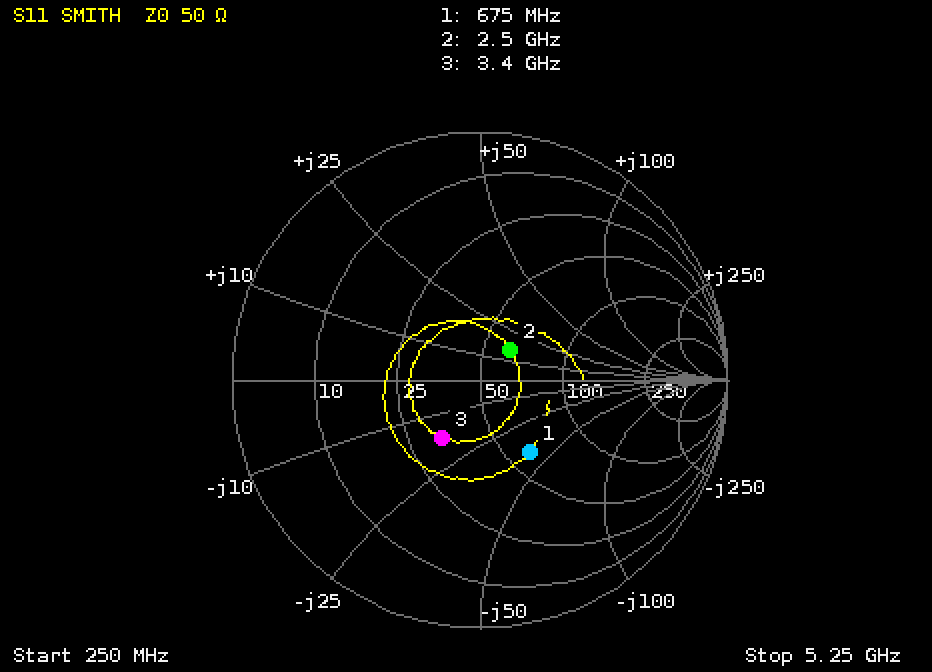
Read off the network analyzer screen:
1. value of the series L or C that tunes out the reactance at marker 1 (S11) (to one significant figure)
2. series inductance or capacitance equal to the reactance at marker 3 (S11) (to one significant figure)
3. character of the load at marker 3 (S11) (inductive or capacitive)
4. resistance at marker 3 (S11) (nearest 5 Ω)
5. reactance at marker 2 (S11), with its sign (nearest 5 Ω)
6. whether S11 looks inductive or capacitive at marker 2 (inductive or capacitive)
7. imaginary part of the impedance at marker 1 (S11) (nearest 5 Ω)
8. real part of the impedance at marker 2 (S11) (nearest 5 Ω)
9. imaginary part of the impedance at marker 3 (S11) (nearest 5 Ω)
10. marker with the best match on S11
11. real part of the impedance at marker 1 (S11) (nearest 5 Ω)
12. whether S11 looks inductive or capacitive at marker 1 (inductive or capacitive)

9 nH
3 pF
capacitive
35 Ω
+15 Ω
inductive
-40 Ω
60 Ω
-15 Ω
marker 2
60 Ω
capacitive
